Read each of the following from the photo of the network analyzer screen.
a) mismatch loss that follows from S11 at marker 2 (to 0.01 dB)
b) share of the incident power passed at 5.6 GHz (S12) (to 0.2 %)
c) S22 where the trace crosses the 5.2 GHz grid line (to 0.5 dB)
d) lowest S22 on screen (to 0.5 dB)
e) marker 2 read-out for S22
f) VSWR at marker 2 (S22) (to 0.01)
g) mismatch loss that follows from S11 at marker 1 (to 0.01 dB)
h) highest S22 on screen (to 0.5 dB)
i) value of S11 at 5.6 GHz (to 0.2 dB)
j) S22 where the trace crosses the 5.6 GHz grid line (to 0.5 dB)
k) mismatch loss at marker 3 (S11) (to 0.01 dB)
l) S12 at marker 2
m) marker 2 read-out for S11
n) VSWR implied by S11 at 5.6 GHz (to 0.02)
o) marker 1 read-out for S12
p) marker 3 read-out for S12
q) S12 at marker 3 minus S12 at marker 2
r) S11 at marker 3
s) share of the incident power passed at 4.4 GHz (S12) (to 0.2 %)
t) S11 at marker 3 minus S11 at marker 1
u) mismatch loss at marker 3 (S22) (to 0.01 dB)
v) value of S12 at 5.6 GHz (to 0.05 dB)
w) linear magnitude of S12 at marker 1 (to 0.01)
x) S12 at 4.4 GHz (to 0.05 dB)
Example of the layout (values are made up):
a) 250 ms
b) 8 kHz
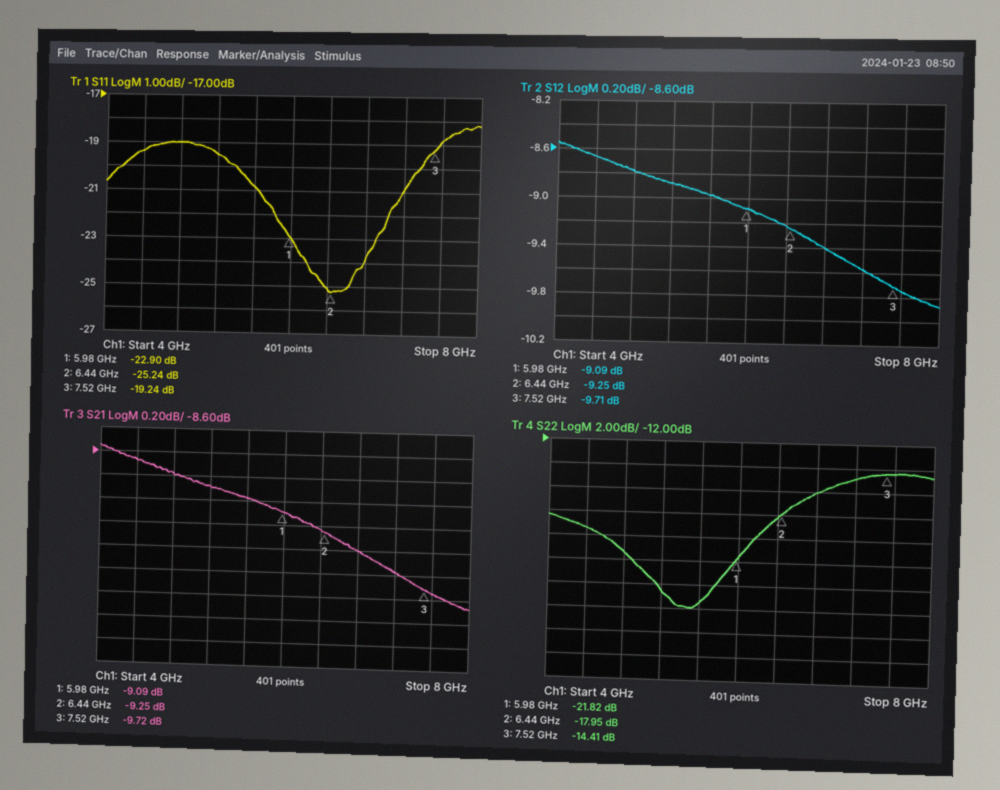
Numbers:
a) 0.01 dB
b) 12.6 %
c) -24.5 dB
d) -26.0 dB
e) -17.95 dB
f) 1.29
g) 0.02 dB
h) -14.5 dB
i) -20.8 dB
j) -25.5 dB
k) 0.05 dB
l) -9.25 dB
m) -25.24 dB
n) 1.20
o) -9.09 dB
p) -9.71 dB
q) -0.46 dB
r) -19.24 dB
s) 13.6 %
t) 3.66 dB
u) 0.16 dB
v) -9.00 dB
w) 0.35
x) -8.65 dB
